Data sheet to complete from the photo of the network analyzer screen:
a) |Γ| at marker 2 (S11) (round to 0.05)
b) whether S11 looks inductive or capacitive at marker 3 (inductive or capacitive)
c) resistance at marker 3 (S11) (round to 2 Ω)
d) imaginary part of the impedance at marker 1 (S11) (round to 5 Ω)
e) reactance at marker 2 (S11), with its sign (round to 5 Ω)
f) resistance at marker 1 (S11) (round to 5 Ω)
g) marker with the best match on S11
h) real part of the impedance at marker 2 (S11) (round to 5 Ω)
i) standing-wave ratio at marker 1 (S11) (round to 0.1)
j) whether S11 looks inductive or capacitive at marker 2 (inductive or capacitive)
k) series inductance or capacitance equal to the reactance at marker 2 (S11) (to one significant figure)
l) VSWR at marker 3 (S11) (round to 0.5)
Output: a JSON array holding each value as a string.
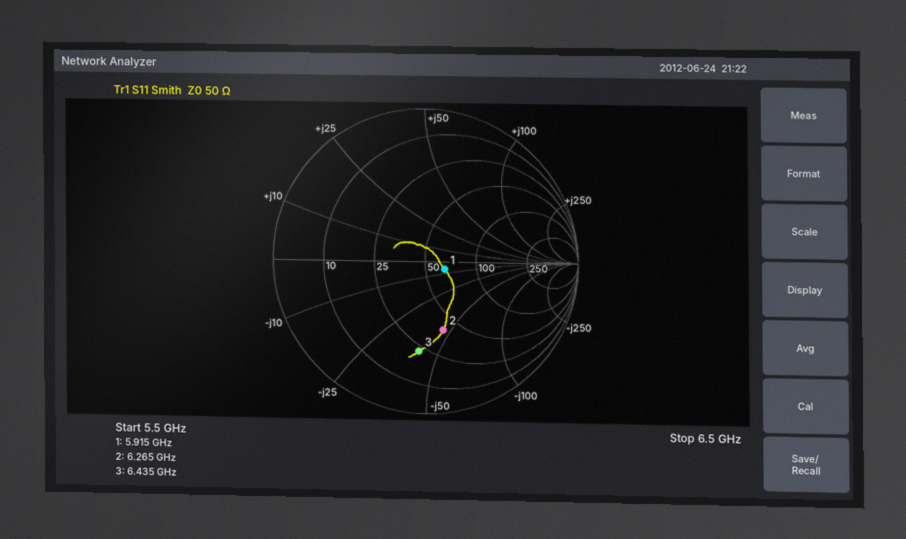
["0.45", "capacitive", "22 Ω", "-5 Ω", "-45 Ω", "65 Ω", "marker 1", "40 Ω", "1.3", "capacitive", "600 fF", "4.0"]
